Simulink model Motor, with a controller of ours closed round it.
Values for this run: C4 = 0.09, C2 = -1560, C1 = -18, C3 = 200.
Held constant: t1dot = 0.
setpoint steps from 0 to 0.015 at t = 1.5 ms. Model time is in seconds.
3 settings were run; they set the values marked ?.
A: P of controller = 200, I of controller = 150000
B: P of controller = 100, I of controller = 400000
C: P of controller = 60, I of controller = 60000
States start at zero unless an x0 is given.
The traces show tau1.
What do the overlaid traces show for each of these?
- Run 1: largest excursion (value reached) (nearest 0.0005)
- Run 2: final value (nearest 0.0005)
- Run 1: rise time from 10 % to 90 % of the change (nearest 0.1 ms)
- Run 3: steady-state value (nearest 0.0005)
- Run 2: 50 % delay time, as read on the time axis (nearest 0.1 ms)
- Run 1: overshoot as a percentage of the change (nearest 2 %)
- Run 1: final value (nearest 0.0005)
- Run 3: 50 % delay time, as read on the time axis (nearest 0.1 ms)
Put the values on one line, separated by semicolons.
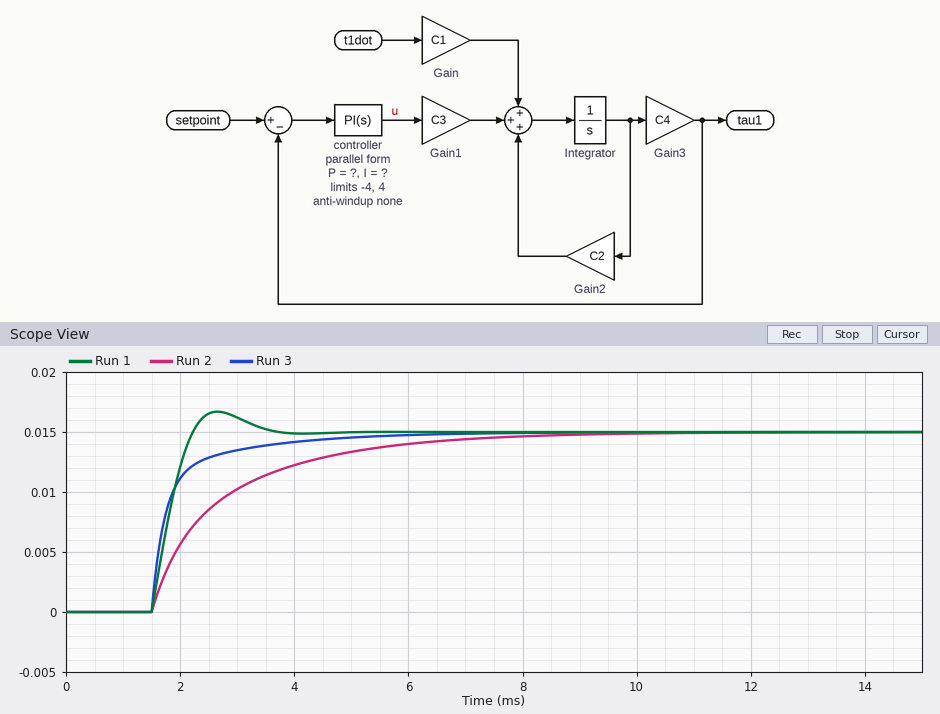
0.0165; 0.0150; 0.5 ms; 0.0150; 2.3 ms; 12 %; 0.0150; 1.7 ms
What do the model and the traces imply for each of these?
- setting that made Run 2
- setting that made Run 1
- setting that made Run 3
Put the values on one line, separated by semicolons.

C; B; A
